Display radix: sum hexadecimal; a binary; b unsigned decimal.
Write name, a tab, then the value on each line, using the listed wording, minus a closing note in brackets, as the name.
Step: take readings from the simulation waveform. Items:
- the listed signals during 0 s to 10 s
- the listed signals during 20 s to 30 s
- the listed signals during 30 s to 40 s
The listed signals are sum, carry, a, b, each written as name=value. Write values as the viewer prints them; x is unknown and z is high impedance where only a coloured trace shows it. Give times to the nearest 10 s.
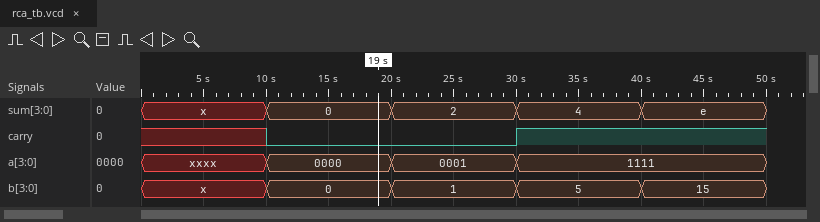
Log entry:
the listed signals during 0 s to 10 s	sum=x, carry=x, a=xxxx, b=x
the listed signals during 20 s to 30 s	sum=2, carry=0, a=0001, b=1
the listed signals during 30 s to 40 s	sum=4, carry=1, a=1111, b=5
